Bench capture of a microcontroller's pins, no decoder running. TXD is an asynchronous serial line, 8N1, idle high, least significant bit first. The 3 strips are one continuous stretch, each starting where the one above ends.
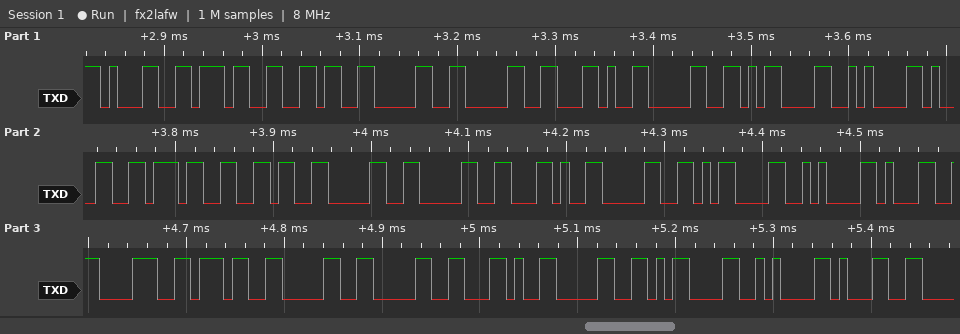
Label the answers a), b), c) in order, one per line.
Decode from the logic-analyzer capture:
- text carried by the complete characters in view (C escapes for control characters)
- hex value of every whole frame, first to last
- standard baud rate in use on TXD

a) "17600,0\r\n17600,0\r\n18700,0\r\n1"
b) 0x31 0x37 0x36 0x30 0x30 0x2C 0x30 0x0D 0x0A 0x31 0x37 0x36 0x30 0x30 0x2C 0x30 0x0D 0x0A 0x31 0x38 0x37 0x30 0x30 0x2C 0x30 0x0D 0x0A 0x31
c) 115200 baud
